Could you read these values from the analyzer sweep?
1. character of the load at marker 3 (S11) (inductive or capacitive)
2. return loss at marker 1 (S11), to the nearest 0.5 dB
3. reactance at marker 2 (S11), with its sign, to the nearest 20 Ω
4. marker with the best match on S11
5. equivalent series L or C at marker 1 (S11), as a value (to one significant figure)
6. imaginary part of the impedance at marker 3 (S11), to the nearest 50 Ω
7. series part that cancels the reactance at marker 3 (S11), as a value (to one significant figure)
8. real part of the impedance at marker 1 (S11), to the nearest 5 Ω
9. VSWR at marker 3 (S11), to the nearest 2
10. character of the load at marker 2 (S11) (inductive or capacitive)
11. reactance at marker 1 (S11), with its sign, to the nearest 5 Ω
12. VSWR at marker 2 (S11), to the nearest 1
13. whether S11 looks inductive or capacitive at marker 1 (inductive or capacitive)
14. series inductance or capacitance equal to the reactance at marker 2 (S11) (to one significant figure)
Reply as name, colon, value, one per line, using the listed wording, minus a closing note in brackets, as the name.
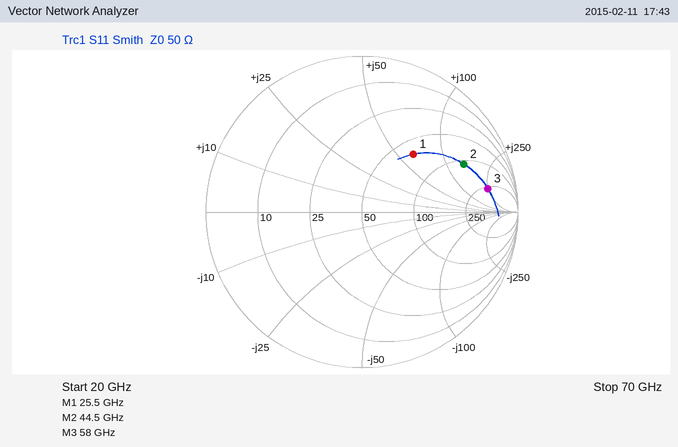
character of the load at marker 3 (S11): inductive
return loss at marker 1 (S11), to the nearest 0.5 dB: 6.0 dB
reactance at marker 2 (S11), with its sign, to the nearest 20 Ω: +140 Ω
marker with the best match on S11: marker 1
equivalent series L or C at marker 1 (S11), as a value: 400 pH
imaginary part of the impedance at marker 3 (S11), to the nearest 50 Ω: +250 Ω
series part that cancels the reactance at marker 3 (S11), as a value: 10 fF
real part of the impedance at marker 1 (S11), to the nearest 5 Ω: 65 Ω
VSWR at marker 3 (S11), to the nearest 2: 10
character of the load at marker 2 (S11): inductive
reactance at marker 1 (S11), with its sign, to the nearest 5 Ω: +65 Ω
VSWR at marker 2 (S11), to the nearest 1: 6
whether S11 looks inductive or capacitive at marker 1: inductive
series inductance or capacitance equal to the reactance at marker 2 (S11): 500 pH
